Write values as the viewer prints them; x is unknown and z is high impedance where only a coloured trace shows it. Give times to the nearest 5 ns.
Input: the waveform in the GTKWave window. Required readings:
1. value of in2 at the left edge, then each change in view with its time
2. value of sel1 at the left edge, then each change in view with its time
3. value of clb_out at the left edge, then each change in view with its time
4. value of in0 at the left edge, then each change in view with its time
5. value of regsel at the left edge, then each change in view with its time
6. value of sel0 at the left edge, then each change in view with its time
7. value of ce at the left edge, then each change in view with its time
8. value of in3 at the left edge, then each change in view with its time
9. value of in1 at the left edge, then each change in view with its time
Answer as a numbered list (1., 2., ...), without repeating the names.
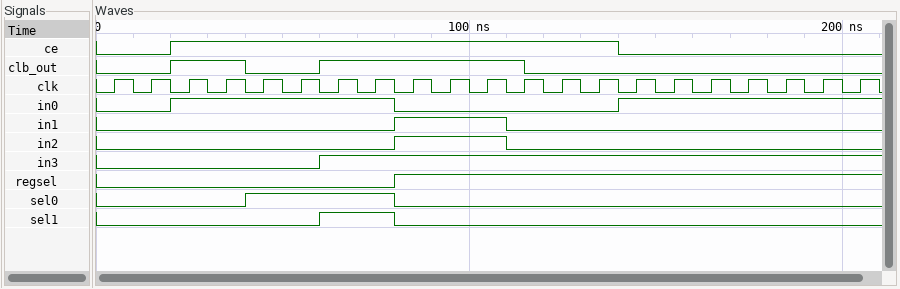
1. 0, 1 at 80 ns, 0 at 110 ns
2. 0, 1 at 60 ns, 0 at 80 ns
3. 0, 1 at 20 ns, 0 at 40 ns, 1 at 60 ns, 0 at 115 ns
4. 0, 1 at 20 ns, 0 at 80 ns, 1 at 140 ns
5. 0, 1 at 80 ns
6. 0, 1 at 40 ns, 0 at 80 ns
7. 0, 1 at 20 ns, 0 at 140 ns
8. 0, 1 at 60 ns
9. 0, 1 at 80 ns, 0 at 110 ns
